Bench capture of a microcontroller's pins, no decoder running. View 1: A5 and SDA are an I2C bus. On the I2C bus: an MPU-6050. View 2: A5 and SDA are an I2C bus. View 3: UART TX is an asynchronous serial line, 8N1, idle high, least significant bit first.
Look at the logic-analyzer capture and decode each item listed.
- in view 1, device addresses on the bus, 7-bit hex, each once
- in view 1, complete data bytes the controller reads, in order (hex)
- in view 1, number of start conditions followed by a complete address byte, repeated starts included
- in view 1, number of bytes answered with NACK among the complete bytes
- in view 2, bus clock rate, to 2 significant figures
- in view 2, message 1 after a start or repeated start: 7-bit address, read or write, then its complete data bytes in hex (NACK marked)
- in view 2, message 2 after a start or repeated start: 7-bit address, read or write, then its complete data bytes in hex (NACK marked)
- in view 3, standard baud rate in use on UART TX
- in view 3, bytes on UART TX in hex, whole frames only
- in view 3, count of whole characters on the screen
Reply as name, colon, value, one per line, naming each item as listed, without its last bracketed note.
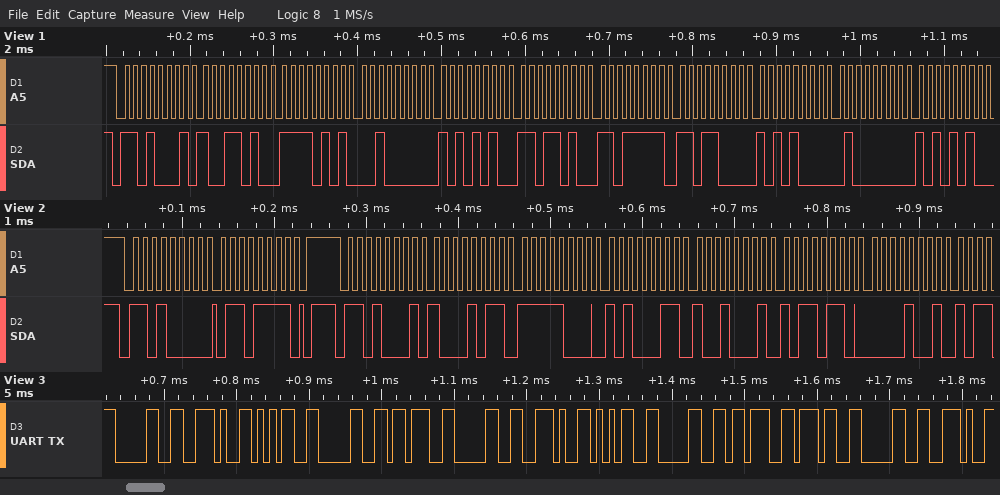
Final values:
in view 1, device addresses on the bus, 7-bit hex, each once: 0x68
in view 1, complete data bytes the controller reads, in order: 9A F5 20 AA DA DF D8 A8 40 AA
in view 1, number of start conditions followed by a complete address byte, repeated starts included: 1
in view 1, number of bytes answered with NACK among the complete bytes: 0
in view 2, bus clock rate, to 2 significant figures: 100 kHz
in view 2, message 1 after a start or repeated start: 7-bit address, read or write, then its complete data bytes in hex: 0x68 write: 6F
in view 2, message 2 after a start or repeated start: 7-bit address, read or write, then its complete data bytes in hex: 0x68 read: 8B F8 A3 91 B6 09
in view 3, standard baud rate in use on UART TX: 115200 baud
in view 3, bytes on UART TX in hex, whole frames only: 30 2E 35 30 3B 30 2E 35 30 3B 37 30 2E
in view 3, count of whole characters on the screen: 13
